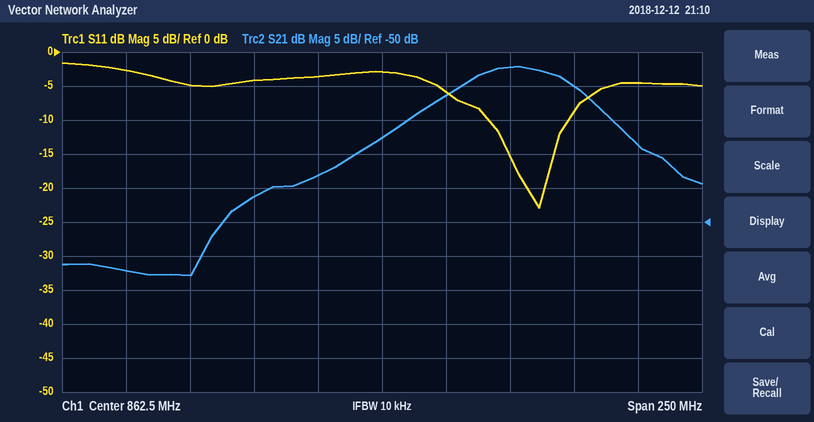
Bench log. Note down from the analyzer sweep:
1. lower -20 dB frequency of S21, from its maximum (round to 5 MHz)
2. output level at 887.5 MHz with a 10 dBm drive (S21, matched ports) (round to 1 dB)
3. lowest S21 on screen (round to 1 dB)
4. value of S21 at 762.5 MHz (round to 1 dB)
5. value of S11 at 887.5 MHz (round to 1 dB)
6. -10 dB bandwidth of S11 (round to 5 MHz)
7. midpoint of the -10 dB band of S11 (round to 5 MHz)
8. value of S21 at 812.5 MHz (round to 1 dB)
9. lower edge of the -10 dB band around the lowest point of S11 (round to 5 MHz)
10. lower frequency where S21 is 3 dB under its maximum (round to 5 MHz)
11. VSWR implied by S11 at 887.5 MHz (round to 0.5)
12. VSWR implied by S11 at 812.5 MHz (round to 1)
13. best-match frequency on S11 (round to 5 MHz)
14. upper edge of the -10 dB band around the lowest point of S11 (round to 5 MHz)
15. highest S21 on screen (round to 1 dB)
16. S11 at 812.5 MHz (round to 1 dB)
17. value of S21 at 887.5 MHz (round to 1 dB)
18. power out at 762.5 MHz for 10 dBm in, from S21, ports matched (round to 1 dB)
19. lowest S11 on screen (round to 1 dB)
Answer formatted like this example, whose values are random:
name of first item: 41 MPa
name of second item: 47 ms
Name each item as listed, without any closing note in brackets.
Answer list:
lower -20 dB frequency of S21, from its maximum: 810 MHz
output level at 887.5 MHz with a 10 dBm drive (S21, matched ports): -21 dBm
lowest S21 on screen: -58 dB
value of S21 at 762.5 MHz: -57 dB
value of S11 at 887.5 MHz: -6 dB
-10 dB bandwidth of S11: 30 MHz
midpoint of the -10 dB band of S11: 920 MHz
value of S21 at 812.5 MHz: -46 dB
lower edge of the -10 dB band around the lowest point of S11: 905 MHz
lower frequency where S21 is 3 dB under its maximum: 895 MHz
VSWR implied by S11 at 887.5 MHz: 3.0
VSWR implied by S11 at 812.5 MHz: 4
best-match frequency on S11: 925 MHz
upper edge of the -10 dB band around the lowest point of S11: 935 MHz
highest S21 on screen: -27 dB
S11 at 812.5 MHz: -4 dB
value of S21 at 887.5 MHz: -31 dB
power out at 762.5 MHz for 10 dBm in, from S21, ports matched: -47 dBm
lowest S11 on screen: -23 dB
